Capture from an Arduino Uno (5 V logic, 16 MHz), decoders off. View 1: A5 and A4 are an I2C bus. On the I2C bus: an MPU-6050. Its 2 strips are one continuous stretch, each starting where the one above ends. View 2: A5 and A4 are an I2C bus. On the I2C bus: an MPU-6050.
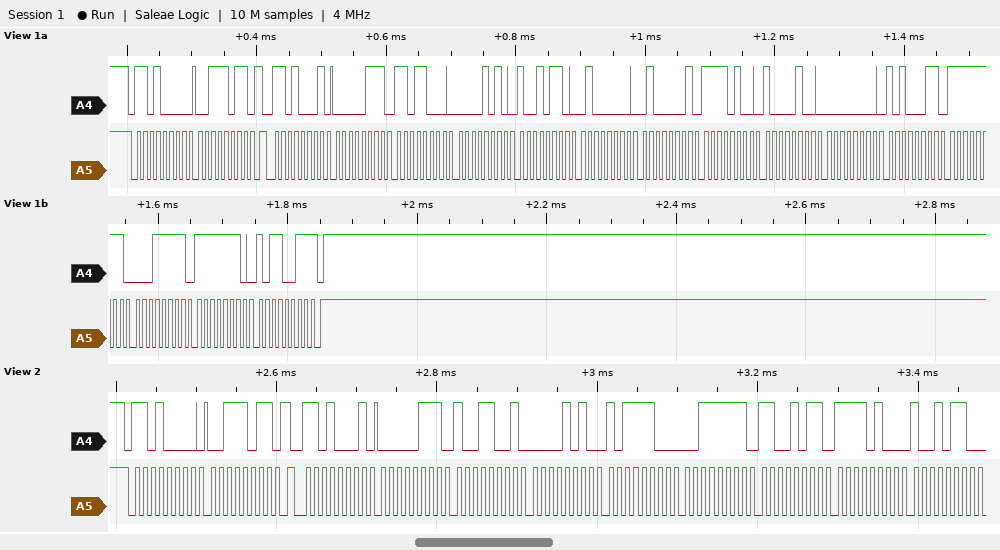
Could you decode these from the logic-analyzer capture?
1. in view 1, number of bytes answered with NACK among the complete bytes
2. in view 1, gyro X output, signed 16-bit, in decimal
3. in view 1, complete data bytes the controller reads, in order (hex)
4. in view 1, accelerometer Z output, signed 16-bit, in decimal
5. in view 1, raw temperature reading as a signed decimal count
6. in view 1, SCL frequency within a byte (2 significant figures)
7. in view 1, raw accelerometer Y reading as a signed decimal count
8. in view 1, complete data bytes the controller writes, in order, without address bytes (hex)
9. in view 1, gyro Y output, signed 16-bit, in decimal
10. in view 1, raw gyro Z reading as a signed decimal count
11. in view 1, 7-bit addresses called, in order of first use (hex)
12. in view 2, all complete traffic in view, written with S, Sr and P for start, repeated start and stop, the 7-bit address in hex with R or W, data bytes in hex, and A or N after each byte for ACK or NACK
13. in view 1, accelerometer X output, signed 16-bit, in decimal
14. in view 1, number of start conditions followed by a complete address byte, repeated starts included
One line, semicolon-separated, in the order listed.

1; 163; 07 D8 0A 96 40 41 F4 84 00 A3 FF 1F FE B3; 16449; -2940; 100 kHz; 2710; 3B; -225; -333; 0x68; S 68W A 3B A Sr 68R A 07 A 99 A 0A A BC A 3F A CB A F4 A 96 A; 2008; 2
